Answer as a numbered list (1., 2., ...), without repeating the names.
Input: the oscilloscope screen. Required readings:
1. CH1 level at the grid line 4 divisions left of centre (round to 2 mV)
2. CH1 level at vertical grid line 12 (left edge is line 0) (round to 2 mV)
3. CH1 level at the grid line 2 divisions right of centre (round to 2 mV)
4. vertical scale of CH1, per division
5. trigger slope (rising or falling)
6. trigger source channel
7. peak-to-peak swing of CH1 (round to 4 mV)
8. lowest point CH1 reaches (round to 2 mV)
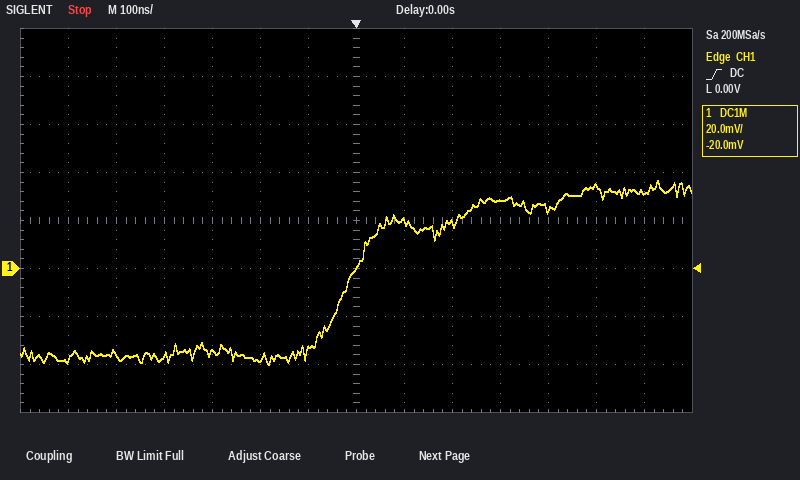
1. -36 mV
2. 34 mV
3. 18 mV
4. 20 mV
5. rising
6. CH1
7. 76 mV
8. -40 mV
